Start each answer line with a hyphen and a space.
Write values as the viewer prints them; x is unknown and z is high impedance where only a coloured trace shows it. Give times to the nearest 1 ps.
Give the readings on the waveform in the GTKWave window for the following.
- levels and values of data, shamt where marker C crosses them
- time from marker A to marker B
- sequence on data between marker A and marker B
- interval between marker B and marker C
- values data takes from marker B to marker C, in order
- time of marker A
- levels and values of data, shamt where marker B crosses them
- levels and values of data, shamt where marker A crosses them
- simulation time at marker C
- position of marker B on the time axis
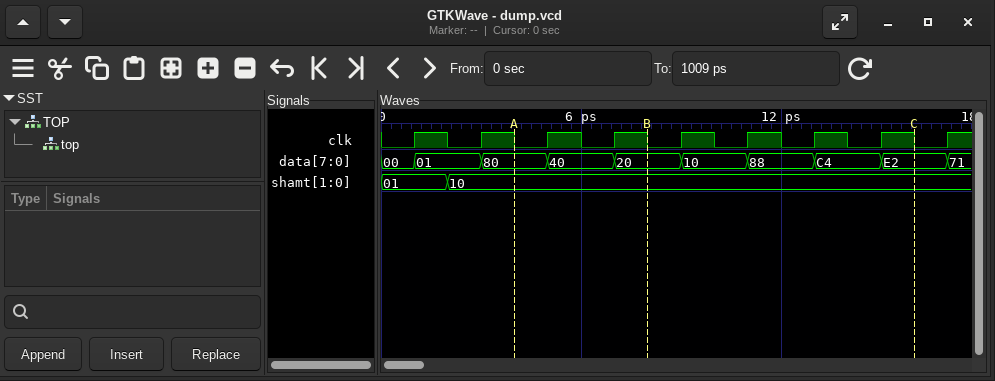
- data=E2, shamt=10
- 4 ps
- 80, 40, 20
- 8 ps
- 20, 10, 88, C4, E2
- 4 ps
- data=20, shamt=10
- data=80, shamt=10
- 16 ps
- 8 ps
